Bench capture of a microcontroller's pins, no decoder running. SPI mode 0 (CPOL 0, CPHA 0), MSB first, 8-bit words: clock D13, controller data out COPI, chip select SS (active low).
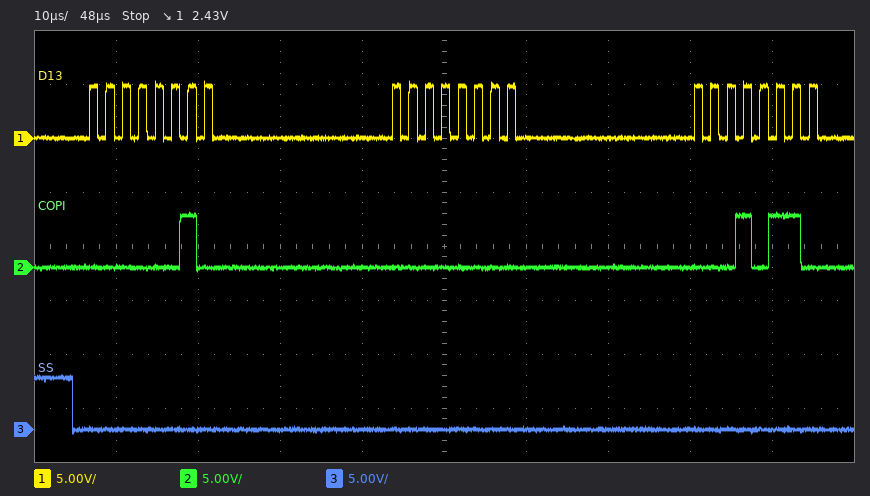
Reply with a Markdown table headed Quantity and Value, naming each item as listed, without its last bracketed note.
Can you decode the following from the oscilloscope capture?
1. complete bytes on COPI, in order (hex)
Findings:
| Quantity | Value |
|---|---|
| complete bytes on COPI, in order | 02 00 16 |
